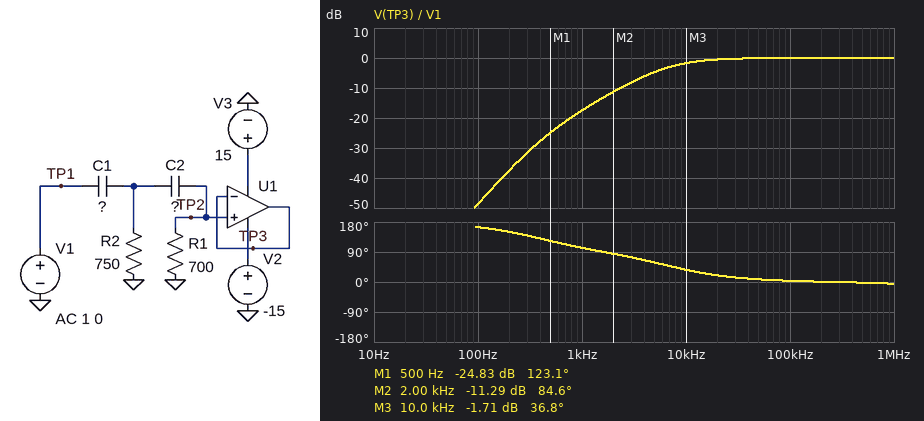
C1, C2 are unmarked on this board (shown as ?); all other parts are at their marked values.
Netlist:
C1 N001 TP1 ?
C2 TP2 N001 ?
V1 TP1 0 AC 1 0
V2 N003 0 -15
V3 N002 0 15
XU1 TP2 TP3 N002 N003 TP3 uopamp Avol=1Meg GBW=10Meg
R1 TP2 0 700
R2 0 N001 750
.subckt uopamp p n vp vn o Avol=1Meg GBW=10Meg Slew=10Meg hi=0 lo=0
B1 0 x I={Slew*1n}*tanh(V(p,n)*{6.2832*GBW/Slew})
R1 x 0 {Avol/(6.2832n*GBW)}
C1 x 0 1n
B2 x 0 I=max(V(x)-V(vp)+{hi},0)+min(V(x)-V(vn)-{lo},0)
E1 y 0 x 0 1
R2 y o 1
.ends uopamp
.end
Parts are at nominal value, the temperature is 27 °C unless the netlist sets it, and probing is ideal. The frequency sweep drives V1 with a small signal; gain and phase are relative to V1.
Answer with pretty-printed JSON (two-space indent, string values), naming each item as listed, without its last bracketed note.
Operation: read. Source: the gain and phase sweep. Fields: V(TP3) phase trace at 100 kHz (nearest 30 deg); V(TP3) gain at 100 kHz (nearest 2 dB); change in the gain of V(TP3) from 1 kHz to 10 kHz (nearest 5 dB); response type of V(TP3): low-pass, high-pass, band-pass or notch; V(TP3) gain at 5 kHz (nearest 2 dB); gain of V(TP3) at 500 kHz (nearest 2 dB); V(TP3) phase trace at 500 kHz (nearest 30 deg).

{
  "V(TP3) phase trace at 100 kHz": "0 deg",
  "V(TP3) gain at 100 kHz": "0 dB",
  "change in the gain of V(TP3) from 1 kHz to 10 kHz": "15 dB",
  "response type of V(TP3): low-pass, high-pass, band-pass or notch": "high-pass",
  "V(TP3) gain at 5 kHz": "-4 dB",
  "gain of V(TP3) at 500 kHz": "0 dB",
  "V(TP3) phase trace at 500 kHz": "0 deg"
}
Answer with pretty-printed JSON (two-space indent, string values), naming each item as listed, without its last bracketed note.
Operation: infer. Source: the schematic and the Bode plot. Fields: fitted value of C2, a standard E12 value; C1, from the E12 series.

{
  "fitted value of C2, a standard E12 value": "270 nF",
  "C1, from the E12 series": "68 nF"
}
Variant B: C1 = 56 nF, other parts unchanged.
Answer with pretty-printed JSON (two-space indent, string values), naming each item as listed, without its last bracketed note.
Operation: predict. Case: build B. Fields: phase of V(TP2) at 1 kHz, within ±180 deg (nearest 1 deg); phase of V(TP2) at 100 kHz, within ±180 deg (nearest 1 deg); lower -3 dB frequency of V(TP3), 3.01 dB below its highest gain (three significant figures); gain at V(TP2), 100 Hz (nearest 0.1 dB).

{
  "phase of V(TP2) at 1 kHz, within ±180 deg": "104 deg",
  "phase of V(TP2) at 100 kHz, within ±180 deg": "5 deg",
  "lower -3 dB frequency of V(TP3), 3.01 dB below its highest gain": "8.31 kHz",
  "gain at V(TP2), 100 Hz": "-50.4 dB"
}
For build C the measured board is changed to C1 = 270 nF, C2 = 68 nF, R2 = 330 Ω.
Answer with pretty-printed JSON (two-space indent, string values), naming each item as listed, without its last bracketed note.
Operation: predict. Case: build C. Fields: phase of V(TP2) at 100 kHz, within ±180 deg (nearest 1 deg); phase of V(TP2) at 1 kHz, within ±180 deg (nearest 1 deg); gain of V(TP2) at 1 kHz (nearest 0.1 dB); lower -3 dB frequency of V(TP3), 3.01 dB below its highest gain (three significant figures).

{
  "phase of V(TP2) at 100 kHz, within ±180 deg": "3 deg",
  "phase of V(TP2) at 1 kHz, within ±180 deg": "130 deg",
  "gain of V(TP2) at 1 kHz": "-17.8 dB",
  "lower -3 dB frequency of V(TP3), 3.01 dB below its highest gain": "5.01 kHz"
}
